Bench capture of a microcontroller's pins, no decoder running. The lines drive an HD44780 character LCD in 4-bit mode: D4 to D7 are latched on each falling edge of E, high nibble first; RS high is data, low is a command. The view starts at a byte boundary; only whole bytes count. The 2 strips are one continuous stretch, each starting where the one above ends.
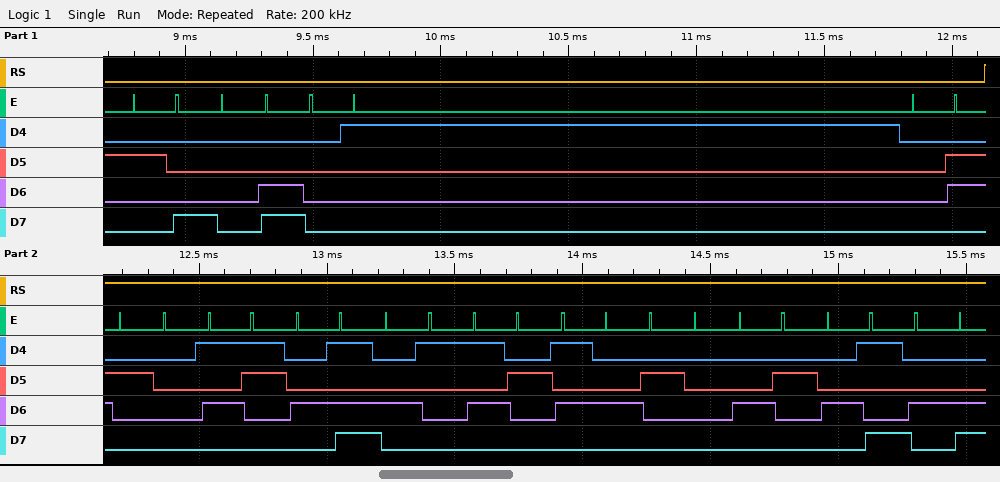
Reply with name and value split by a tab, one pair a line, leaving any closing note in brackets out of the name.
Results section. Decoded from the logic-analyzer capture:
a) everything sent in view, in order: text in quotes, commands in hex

everything sent in view, in order: text in quotes, commands in hex	0x28 0x0C 0x01 0x06 " SMART BIL"
